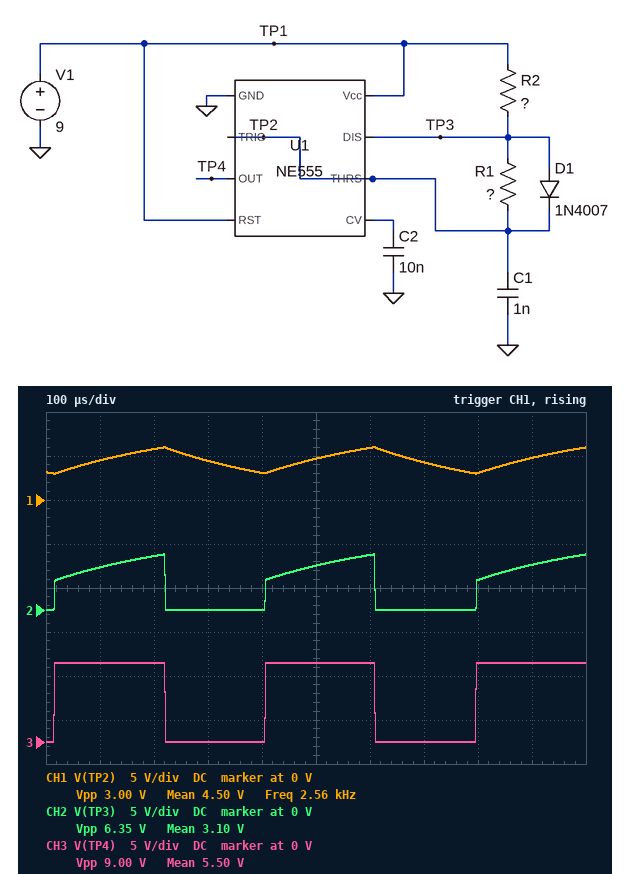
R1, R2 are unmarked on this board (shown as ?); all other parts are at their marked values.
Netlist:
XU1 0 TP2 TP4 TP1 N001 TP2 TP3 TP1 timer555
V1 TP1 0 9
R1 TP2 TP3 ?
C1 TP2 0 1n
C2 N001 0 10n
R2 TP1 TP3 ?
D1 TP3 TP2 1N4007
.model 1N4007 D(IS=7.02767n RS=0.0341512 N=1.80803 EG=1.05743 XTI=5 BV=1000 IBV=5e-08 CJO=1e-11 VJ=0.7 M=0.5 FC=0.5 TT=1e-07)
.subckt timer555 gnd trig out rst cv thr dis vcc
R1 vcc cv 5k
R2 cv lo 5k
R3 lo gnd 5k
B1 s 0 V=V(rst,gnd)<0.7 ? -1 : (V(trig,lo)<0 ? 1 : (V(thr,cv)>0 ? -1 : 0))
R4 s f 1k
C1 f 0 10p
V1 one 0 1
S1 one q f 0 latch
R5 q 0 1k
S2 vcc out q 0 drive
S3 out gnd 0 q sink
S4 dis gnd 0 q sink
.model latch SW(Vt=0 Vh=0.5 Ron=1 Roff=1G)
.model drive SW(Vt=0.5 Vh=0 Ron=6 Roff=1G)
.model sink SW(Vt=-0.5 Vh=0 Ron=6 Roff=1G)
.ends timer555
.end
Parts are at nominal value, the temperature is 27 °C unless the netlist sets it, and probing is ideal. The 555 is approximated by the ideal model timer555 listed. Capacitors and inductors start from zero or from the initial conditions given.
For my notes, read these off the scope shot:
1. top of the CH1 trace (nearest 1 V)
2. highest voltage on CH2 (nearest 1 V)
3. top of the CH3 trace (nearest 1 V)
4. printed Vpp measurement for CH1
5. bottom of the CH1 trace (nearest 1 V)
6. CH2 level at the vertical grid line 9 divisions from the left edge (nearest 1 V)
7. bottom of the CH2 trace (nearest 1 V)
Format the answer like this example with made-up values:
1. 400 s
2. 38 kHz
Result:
1. 6 V
2. 6 V
3. 9 V
4. 3.00 V
5. 3 V
6. 5 V
7. 0 V
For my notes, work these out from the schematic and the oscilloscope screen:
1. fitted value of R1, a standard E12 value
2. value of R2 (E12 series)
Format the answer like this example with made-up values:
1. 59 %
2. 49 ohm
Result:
1. 270 kΩ
2. 270 kΩ
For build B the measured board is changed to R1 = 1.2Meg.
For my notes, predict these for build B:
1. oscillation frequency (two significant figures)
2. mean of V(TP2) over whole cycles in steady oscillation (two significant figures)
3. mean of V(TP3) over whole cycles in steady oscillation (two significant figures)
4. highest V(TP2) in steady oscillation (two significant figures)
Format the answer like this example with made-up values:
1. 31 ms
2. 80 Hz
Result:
1. 970 Hz
2. 4.4 V
3. 1.0 V
4. 6.0 V
